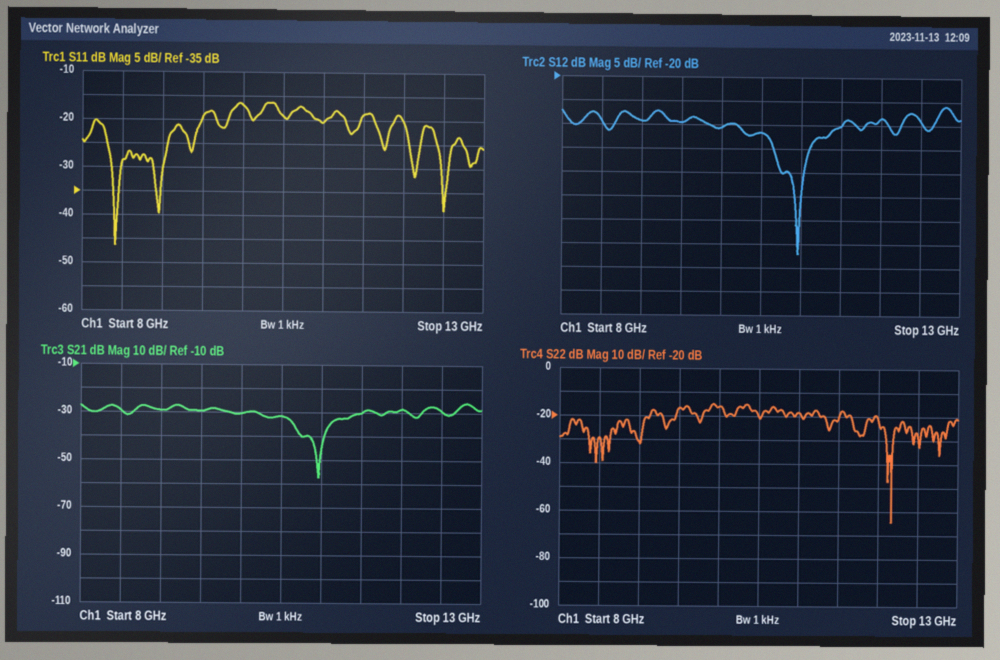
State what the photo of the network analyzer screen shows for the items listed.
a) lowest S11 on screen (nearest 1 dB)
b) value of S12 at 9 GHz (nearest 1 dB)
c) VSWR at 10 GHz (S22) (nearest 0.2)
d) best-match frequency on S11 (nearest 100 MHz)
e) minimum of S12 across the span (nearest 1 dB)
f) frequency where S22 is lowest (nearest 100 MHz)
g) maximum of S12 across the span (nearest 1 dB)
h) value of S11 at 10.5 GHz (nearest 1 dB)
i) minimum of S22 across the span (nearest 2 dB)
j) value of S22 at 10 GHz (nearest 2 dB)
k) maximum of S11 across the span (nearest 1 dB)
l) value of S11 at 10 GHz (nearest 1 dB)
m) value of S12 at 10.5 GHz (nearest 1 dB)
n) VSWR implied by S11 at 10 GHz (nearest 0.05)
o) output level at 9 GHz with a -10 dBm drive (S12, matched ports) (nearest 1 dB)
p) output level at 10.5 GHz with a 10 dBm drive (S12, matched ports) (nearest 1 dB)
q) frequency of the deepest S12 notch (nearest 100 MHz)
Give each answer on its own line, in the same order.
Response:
-46 dB
-29 dB
1.4
8.4 GHz
-57 dB
12.2 GHz
-26 dB
-19 dB
-64 dB
-16 dB
-16 dB
-17 dB
-32 dB
1.35
-39 dBm
-22 dBm
11.0 GHz
